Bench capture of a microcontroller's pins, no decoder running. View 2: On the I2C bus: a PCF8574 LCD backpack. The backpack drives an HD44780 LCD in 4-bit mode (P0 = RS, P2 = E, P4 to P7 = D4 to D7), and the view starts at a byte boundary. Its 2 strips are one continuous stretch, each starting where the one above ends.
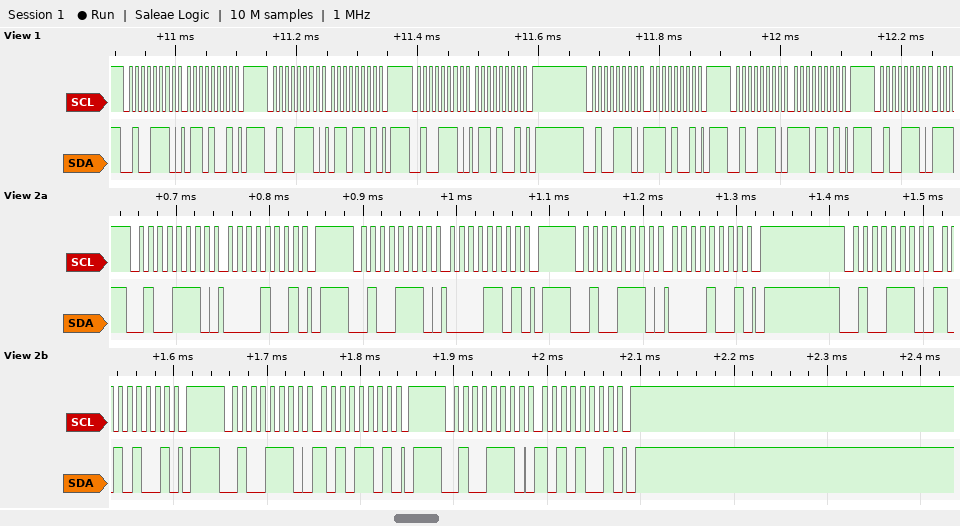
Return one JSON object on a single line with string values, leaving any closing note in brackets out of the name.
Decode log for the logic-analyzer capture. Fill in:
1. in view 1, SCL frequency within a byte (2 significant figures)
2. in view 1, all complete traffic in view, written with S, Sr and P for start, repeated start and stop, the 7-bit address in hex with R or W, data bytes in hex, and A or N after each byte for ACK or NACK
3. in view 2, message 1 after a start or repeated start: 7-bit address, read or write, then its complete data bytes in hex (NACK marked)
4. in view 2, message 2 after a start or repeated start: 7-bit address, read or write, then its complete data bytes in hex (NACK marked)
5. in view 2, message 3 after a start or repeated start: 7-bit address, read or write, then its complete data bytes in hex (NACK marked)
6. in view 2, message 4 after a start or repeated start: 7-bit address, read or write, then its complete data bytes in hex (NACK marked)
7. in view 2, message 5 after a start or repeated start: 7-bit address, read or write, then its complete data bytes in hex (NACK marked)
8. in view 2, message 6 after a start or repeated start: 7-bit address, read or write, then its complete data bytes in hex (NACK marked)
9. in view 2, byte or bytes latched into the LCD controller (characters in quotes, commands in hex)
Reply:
{"in view 1, SCL frequency within a byte": "100 kHz", "in view 1, all complete traffic in view, written with S, Sr and P for start, repeated start and stop, the 7-bit address in hex with R or W, data bytes in hex, and A or N after each byte for ACK or NACK": "S 27W A 69 A P S 27W A 6D A P S 27W A 69 A P S 27W A E9 A P S 27W A ED A P S 27W A", "in view 2, message 1 after a start or repeated start: 7-bit address, read or write, then its complete data bytes in hex": "0x27 write: 09", "in view 2, message 2 after a start or repeated start: 7-bit address, read or write, then its complete data bytes in hex": "0x27 write: 0D", "in view 2, message 3 after a start or repeated start: 7-bit address, read or write, then its complete data bytes in hex": "0x27 write: 09", "in view 2, message 4 after a start or repeated start: 7-bit address, read or write, then its complete data bytes in hex": "0x27 write: A9", "in view 2, message 5 after a start or repeated start: 7-bit address, read or write, then its complete data bytes in hex": "0x27 write: AD", "in view 2, message 6 after a start or repeated start: 7-bit address, read or write, then its complete data bytes in hex": "0x27 write: A9", "in view 2, byte or bytes latched into the LCD controller": "data 0x0A"}
